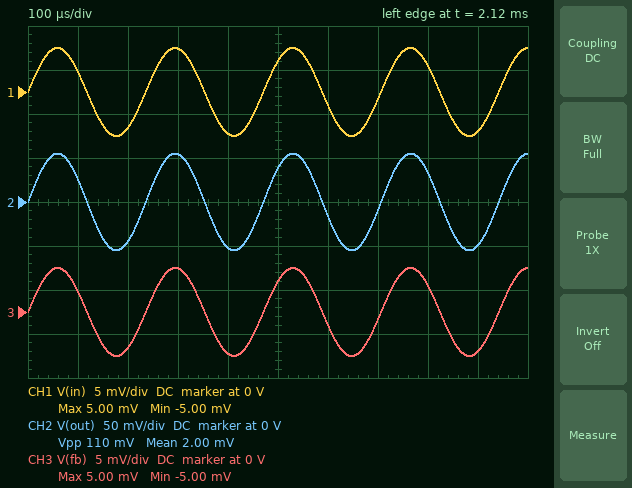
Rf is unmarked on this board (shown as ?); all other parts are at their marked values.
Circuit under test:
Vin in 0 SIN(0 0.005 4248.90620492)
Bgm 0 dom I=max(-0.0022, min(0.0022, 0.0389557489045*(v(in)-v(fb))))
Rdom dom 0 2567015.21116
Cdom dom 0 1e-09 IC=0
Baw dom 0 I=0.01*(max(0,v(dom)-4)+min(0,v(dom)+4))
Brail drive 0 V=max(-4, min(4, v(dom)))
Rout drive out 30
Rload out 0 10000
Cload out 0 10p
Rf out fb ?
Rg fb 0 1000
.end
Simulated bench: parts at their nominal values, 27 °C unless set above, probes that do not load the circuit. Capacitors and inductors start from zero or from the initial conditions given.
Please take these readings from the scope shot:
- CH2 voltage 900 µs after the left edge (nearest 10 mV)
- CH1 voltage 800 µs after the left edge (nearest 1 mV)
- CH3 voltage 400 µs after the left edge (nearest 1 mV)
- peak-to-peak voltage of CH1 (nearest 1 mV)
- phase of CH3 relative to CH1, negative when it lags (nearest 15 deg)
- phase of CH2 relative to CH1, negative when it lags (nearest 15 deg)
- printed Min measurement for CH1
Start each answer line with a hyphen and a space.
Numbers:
- -50 mV
- 3 mV
- -5 mV
- 10 mV
- 0 deg
- 0 deg
- -5.00 mV
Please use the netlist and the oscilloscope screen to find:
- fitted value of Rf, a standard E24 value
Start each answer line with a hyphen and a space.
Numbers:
- 10 kΩ
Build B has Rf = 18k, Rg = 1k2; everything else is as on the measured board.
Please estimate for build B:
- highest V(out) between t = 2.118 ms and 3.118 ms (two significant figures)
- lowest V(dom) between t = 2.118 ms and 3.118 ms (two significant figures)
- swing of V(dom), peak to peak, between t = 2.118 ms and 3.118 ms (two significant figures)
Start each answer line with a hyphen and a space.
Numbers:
- 80 mV
- -80 mV
- 160 mV
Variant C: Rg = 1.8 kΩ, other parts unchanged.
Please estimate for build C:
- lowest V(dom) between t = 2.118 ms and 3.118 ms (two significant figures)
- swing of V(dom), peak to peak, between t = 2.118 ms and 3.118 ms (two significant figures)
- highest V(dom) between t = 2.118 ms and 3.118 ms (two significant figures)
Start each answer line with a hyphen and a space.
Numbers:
- -33 mV
- 66 mV
- 33 mV
